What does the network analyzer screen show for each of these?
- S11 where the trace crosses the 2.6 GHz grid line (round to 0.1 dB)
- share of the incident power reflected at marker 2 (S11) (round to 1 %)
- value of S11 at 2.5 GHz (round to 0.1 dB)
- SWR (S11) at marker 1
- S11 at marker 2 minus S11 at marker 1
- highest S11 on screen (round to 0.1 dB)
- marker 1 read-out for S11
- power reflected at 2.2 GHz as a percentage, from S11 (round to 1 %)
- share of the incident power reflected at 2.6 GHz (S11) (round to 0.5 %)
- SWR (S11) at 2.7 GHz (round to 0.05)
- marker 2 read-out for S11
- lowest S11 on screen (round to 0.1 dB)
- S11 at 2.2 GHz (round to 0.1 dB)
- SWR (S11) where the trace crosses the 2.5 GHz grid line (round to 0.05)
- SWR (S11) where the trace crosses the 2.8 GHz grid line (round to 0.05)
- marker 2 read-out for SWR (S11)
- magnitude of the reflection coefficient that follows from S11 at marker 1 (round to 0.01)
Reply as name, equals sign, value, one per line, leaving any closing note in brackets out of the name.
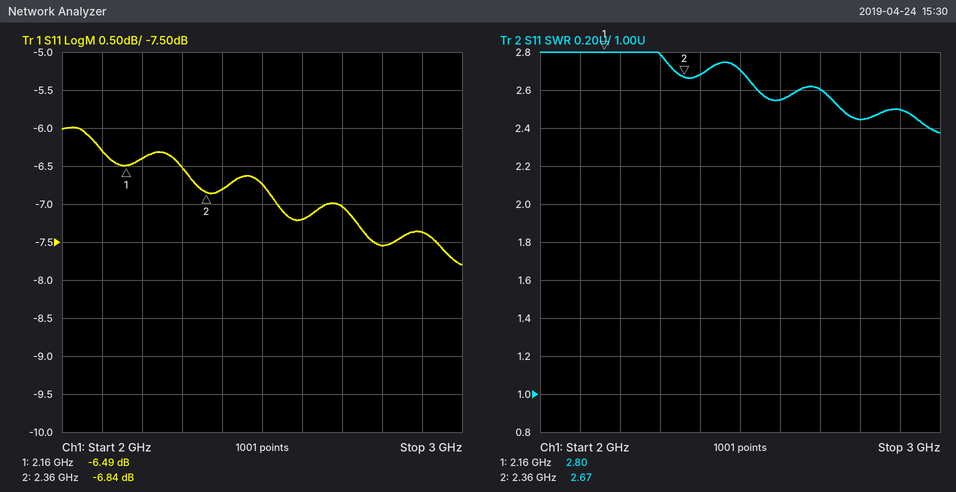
S11 where the trace crosses the 2.6 GHz grid line = -7.2 dB
share of the incident power reflected at marker 2 (S11) = 21 %
value of S11 at 2.5 GHz = -6.7 dB
SWR (S11) at marker 1 = 2.80
S11 at marker 2 minus S11 at marker 1 = -0.35 dB
highest S11 on screen = -6.0 dB
marker 1 read-out for S11 = -6.49 dB
power reflected at 2.2 GHz as a percentage, from S11 = 23 %
share of the incident power reflected at 2.6 GHz (S11) = 19.0 %
SWR (S11) at 2.7 GHz = 2.60
marker 2 read-out for S11 = -6.84 dB
lowest S11 on screen = -7.8 dB
S11 at 2.2 GHz = -6.4 dB
SWR (S11) where the trace crosses the 2.5 GHz grid line = 2.70
SWR (S11) where the trace crosses the 2.8 GHz grid line = 2.45
marker 2 read-out for SWR = 2.67
magnitude of the reflection coefficient that follows from S11 at marker 1 = 0.47
